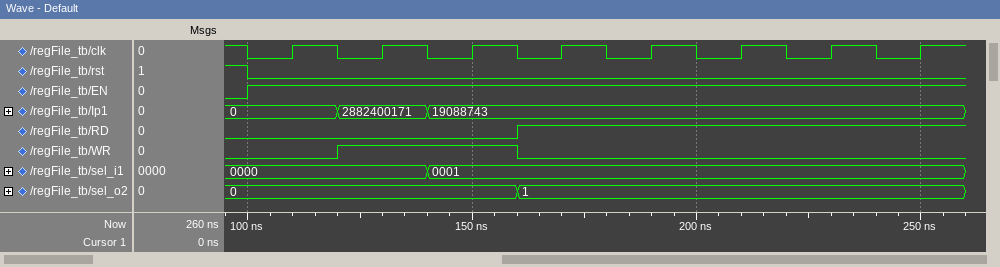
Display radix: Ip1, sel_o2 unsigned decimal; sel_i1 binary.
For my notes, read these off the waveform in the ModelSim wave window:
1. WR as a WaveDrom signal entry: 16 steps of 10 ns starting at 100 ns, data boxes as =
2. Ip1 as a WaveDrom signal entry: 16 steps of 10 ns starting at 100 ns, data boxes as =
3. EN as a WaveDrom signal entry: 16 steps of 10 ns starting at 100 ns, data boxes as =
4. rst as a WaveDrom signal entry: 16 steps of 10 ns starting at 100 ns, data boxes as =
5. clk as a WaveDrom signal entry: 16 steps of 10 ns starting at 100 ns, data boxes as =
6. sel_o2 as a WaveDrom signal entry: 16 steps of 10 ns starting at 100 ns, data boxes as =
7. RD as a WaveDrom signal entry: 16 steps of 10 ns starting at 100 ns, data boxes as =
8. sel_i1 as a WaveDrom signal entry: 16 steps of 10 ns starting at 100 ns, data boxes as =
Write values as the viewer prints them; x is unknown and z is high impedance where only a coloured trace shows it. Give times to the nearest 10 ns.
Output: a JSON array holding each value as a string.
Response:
["{name: 'WR', wave: '0.1...0.........'}", "{name: 'Ip1', wave: '=.=.=...........', data: '0 2882400171 19088743'}", "{name: 'EN', wave: '1...............'}", "{name: 'rst', wave: '0...............'}", "{name: 'clk', wave: '0101010101010101'}", "{name: 'sel_o2', wave: '=.....=.........', data: '0 1'}", "{name: 'RD', wave: '0.....1.........'}", "{name: 'sel_i1', wave: '=...=...........', data: '0000 0001'}"]
